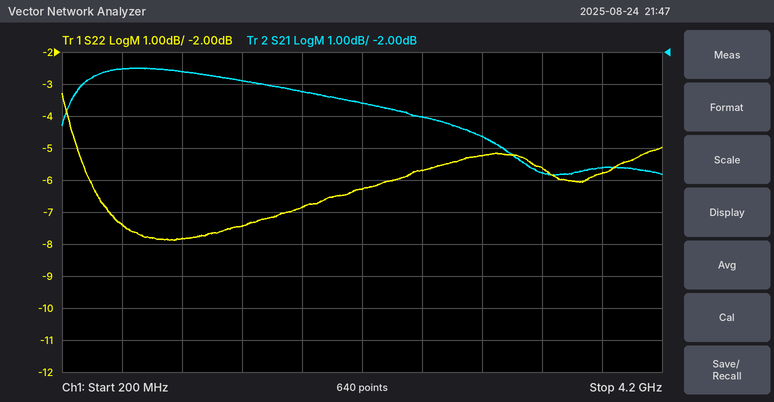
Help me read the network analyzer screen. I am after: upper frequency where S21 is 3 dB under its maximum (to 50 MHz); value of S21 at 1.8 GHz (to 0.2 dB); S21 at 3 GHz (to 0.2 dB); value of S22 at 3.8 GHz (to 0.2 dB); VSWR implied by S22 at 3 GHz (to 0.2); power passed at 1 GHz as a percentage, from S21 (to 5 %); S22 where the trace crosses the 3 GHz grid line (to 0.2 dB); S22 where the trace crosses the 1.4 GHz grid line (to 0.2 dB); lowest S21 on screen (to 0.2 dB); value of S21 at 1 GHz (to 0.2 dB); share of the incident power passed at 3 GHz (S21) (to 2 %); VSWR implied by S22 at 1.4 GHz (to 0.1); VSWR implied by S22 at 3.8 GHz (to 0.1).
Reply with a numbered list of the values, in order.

1. 3.30 GHz
2. -3.2 dB
3. -4.6 dB
4. -5.8 dB
5. 3.4
6. 55 %
7. -5.2 dB
8. -7.4 dB
9. -5.8 dB
10. -2.6 dB
11. 34 %
12. 2.5
13. 3.1
